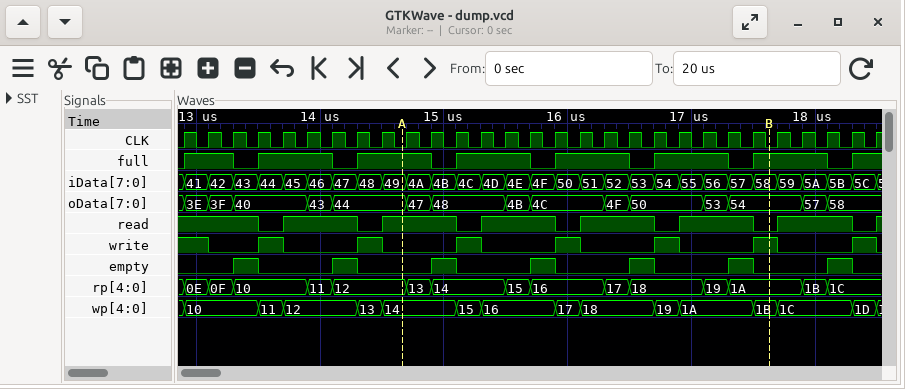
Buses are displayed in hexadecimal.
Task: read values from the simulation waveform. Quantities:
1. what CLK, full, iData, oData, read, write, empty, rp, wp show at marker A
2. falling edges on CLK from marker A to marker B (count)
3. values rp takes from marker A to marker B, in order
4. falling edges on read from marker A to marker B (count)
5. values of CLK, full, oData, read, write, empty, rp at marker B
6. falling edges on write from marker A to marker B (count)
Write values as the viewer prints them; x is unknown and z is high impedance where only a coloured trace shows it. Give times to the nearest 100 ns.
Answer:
CLK=0, full=1, iData=49, oData=44, read=1, write=0, empty=0, rp=12, wp=14
15
12, 13, 14, 15, 16, 17, 18, 19, 1A
4
CLK=0, full=1, oData=54, read=0, write=1, empty=0, rp=1A
3
